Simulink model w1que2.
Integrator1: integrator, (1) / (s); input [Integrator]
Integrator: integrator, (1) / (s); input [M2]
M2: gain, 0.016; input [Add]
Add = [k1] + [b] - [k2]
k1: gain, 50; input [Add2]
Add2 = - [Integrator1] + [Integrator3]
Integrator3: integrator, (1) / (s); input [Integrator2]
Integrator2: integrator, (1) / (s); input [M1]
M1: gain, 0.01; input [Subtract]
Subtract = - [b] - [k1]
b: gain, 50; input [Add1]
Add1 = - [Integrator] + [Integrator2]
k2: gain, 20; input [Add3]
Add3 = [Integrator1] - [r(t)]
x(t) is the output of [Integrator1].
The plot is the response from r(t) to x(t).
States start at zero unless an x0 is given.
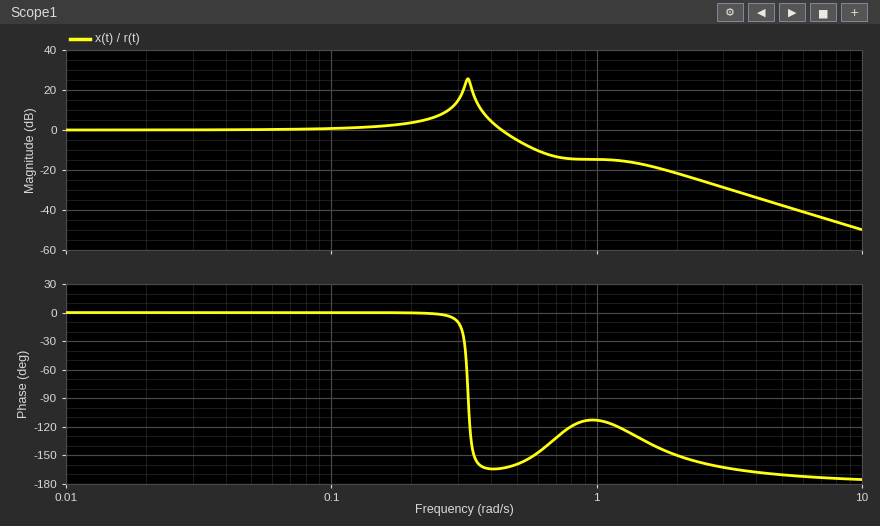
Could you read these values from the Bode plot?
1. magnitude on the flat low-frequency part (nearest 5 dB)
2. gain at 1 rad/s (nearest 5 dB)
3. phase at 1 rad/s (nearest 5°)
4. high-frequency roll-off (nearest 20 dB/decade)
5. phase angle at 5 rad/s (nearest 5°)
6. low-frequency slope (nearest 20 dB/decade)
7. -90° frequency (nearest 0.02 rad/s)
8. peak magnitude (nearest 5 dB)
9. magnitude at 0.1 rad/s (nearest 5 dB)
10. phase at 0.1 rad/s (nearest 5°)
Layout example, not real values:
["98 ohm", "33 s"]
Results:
["0 dB", "-15 dB", "-115°", "-40 dB/decade", "-170°", "0 dB/decade", "0.32 rad/s", "25 dB", "0 dB", "0°"]
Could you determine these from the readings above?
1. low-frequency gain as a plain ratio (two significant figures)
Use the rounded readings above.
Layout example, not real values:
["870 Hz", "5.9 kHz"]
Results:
["1.0"]
